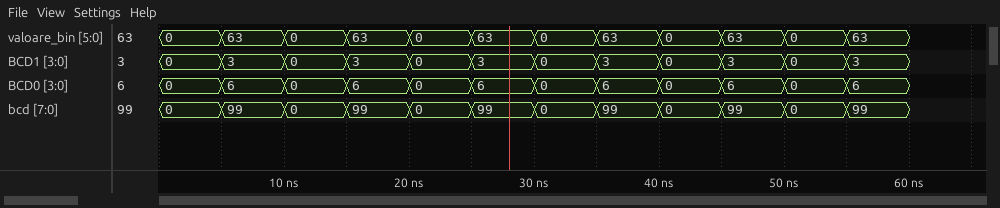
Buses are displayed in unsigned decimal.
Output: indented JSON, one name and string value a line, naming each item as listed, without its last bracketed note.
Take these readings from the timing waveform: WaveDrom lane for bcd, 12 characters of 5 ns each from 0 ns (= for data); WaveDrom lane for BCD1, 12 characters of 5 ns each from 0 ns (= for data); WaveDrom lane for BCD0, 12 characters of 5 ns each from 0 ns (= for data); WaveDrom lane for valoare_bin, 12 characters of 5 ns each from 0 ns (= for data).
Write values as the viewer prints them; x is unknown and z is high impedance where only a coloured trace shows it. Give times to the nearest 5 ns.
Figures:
{
  "WaveDrom lane for bcd, 12 characters of 5 ns each from 0 ns": "{name: 'bcd', wave: '============', data: '0 99 0 99 0 99 0 99 0 99 0 99'}",
  "WaveDrom lane for BCD1, 12 characters of 5 ns each from 0 ns": "{name: 'BCD1', wave: '============', data: '0 3 0 3 0 3 0 3 0 3 0 3'}",
  "WaveDrom lane for BCD0, 12 characters of 5 ns each from 0 ns": "{name: 'BCD0', wave: '============', data: '0 6 0 6 0 6 0 6 0 6 0 6'}",
  "WaveDrom lane for valoare_bin, 12 characters of 5 ns each from 0 ns": "{name: 'valoare_bin', wave: '============', data: '0 63 0 63 0 63 0 63 0 63 0 63'}"
}
